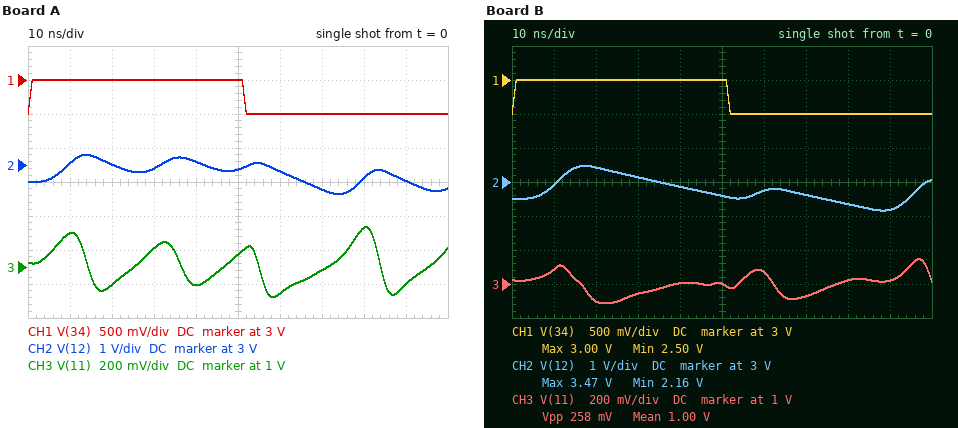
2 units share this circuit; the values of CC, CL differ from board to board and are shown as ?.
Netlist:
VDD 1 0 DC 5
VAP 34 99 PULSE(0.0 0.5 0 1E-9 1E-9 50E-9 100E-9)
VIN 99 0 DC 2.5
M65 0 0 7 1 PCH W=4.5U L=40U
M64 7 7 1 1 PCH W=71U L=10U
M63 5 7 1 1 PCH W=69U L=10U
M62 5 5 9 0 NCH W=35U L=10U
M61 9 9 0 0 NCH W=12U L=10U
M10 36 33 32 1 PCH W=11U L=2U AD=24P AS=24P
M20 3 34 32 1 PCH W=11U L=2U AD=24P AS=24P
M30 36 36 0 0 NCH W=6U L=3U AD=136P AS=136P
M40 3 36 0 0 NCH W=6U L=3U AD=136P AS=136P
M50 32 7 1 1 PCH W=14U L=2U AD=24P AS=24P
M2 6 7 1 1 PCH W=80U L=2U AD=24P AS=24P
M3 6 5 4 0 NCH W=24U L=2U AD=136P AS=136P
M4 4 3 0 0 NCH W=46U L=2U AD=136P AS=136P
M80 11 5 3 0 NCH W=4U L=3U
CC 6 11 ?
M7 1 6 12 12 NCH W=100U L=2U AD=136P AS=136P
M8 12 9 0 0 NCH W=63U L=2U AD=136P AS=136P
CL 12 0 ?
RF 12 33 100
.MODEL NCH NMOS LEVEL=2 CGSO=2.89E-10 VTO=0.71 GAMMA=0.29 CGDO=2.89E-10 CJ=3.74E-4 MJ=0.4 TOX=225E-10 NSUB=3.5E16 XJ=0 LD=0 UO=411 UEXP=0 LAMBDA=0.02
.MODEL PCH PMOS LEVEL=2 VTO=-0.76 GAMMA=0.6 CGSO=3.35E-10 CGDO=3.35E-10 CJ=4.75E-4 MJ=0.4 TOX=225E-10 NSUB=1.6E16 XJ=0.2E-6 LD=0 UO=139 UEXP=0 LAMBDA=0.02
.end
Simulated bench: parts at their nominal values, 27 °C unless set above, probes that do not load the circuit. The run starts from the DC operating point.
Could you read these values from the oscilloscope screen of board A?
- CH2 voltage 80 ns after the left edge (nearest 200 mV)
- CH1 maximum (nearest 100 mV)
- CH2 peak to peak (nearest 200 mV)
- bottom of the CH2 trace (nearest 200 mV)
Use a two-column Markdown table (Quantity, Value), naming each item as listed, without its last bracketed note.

| Quantity | Value |
|---|---|
| CH2 voltage 80 ns after the left edge | 2.6 V |
| CH1 maximum | 3.0 V |
| CH2 peak to peak | 1.2 V |
| bottom of the CH2 trace | 2.2 V |
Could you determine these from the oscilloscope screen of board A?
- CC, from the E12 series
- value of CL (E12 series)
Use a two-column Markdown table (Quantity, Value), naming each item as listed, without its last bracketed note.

| Quantity | Value |
|---|---|
| CC, from the E12 series | 100 fF |
| value of CL | 3.9 pF |
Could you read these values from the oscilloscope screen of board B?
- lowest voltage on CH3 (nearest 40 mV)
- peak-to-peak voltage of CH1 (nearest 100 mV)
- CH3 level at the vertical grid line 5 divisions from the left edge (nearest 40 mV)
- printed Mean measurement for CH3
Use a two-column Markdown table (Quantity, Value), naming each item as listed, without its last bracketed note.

| Quantity | Value |
|---|---|
| lowest voltage on CH3 | 880 mV |
| peak-to-peak voltage of CH1 | 500 mV |
| CH3 level at the vertical grid line 5 divisions from the left edge | 1.00 V |
| printed Mean measurement for CH3 | 1.00 V |
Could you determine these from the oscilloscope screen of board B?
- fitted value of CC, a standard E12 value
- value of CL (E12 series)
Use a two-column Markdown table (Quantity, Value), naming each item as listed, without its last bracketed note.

| Quantity | Value |
|---|---|
| fitted value of CC, a standard E12 value | 68 fF |
| value of CL | 8.2 pF |
